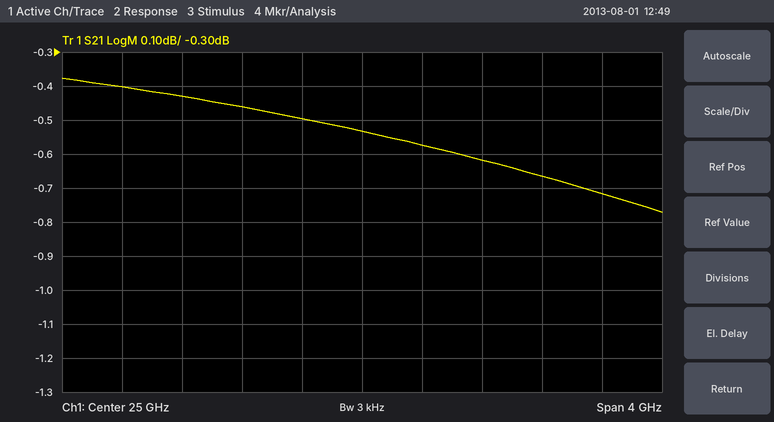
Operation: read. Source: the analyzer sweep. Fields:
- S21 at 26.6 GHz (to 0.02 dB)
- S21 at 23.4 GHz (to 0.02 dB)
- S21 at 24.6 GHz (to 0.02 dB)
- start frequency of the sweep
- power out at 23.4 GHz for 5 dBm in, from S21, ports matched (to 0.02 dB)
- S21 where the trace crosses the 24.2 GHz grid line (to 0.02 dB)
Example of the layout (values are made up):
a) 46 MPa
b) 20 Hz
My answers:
a) -0.72 dB
b) -0.40 dB
c) -0.50 dB
d) 23 GHz
e) 4.60 dBm
f) -0.46 dB
